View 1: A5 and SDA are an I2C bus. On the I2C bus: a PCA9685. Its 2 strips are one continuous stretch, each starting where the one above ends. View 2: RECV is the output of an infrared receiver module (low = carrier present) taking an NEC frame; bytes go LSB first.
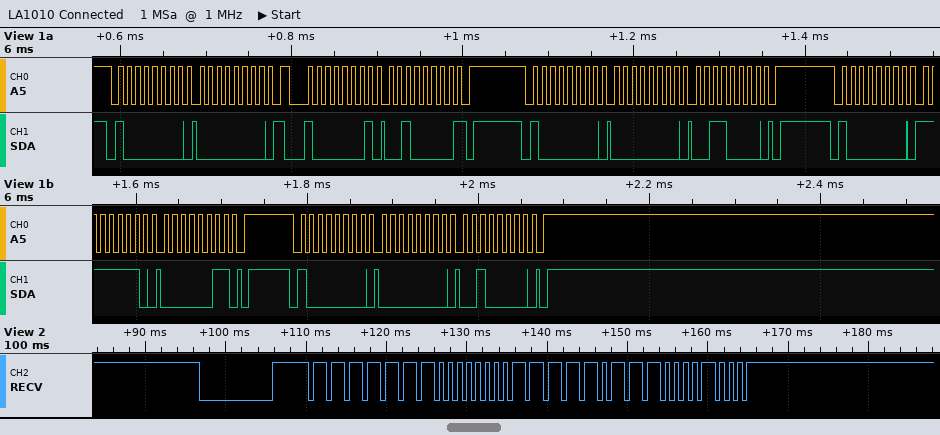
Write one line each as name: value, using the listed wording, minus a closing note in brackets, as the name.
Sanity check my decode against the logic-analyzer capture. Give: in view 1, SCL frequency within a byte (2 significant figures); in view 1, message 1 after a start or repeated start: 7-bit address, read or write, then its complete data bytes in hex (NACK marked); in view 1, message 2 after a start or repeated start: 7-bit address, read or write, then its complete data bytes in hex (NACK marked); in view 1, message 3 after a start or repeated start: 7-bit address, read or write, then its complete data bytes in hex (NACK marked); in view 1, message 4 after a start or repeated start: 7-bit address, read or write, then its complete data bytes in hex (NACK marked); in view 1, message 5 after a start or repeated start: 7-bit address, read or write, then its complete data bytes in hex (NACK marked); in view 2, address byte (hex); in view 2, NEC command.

in view 1, SCL frequency within a byte: 100 kHz
in view 1, message 1 after a start or repeated start: 7-bit address, read or write, then its complete data bytes in hex: 0x40 write: 00
in view 1, message 2 after a start or repeated start: 7-bit address, read or write, then its complete data bytes in hex: 0x40 read: 20 NACK
in view 1, message 3 after a start or repeated start: 7-bit address, read or write, then its complete data bytes in hex: 0x40 write: 00 30
in view 1, message 4 after a start or repeated start: 7-bit address, read or write, then its complete data bytes in hex: 0x40 write: FE 03
in view 1, message 5 after a start or repeated start: 7-bit address, read or write, then its complete data bytes in hex: 0x40 write: 00 20
in view 2, address byte: 0x7F
in view 2, NEC command: 0xEF
